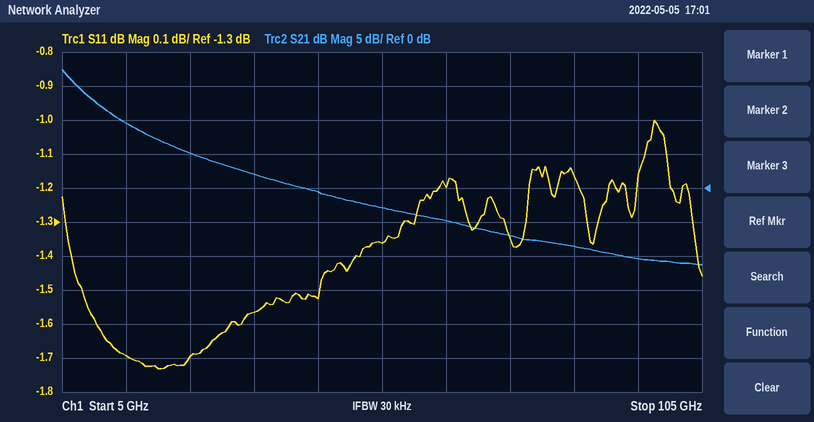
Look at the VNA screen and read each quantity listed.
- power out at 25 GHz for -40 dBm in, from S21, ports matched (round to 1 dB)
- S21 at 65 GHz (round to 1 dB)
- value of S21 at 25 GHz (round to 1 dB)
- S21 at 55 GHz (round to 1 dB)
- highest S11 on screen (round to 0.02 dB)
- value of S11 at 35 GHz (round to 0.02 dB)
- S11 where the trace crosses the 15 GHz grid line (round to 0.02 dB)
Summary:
-35 dBm
-5 dB
5 dB
-3 dB
-1.00 dB
-1.56 dB
-1.70 dB
